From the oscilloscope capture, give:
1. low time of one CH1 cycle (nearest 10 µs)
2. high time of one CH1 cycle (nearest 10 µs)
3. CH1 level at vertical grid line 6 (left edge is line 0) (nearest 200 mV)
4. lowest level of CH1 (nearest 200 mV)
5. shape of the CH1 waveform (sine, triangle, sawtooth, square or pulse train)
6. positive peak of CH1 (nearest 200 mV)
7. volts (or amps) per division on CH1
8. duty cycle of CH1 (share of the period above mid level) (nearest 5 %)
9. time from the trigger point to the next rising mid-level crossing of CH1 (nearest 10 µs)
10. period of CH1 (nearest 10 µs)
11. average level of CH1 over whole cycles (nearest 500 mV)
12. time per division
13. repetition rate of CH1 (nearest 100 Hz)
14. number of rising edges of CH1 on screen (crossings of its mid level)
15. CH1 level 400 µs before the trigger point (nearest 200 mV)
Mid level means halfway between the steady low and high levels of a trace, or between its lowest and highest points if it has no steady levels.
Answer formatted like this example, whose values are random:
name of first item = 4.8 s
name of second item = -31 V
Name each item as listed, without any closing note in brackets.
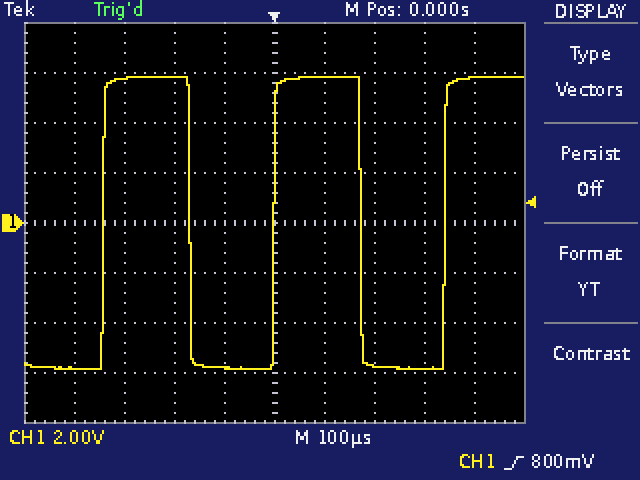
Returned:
low time of one CH1 cycle = 170 µs
high time of one CH1 cycle = 170 µs
CH1 level at vertical grid line 6 (left edge is line 0) = 5.8 V
lowest level of CH1 = -5.8 V
shape of the CH1 waveform = square
positive peak of CH1 = 5.8 V
volts (or amps) per division on CH1 = 2 V
duty cycle of CH1 (share of the period above mid level) = 50 %
time from the trigger point to the next rising mid-level crossing of CH1 = 340 µs
period of CH1 = 340 µs
average level of CH1 over whole cycles = 0.0 V
time per division = 100 µs
repetition rate of CH1 = 2.9 kHz
number of rising edges of CH1 on screen = 3
CH1 level 400 µs before the trigger point = -5.8 V
